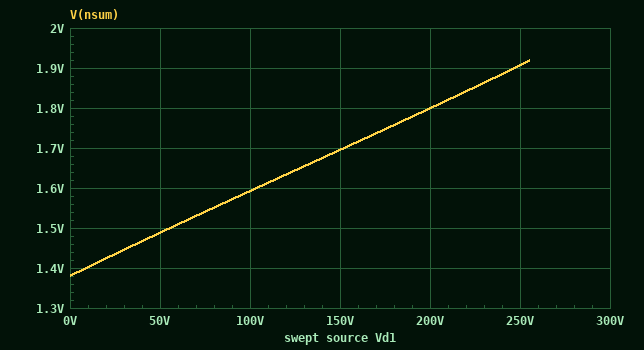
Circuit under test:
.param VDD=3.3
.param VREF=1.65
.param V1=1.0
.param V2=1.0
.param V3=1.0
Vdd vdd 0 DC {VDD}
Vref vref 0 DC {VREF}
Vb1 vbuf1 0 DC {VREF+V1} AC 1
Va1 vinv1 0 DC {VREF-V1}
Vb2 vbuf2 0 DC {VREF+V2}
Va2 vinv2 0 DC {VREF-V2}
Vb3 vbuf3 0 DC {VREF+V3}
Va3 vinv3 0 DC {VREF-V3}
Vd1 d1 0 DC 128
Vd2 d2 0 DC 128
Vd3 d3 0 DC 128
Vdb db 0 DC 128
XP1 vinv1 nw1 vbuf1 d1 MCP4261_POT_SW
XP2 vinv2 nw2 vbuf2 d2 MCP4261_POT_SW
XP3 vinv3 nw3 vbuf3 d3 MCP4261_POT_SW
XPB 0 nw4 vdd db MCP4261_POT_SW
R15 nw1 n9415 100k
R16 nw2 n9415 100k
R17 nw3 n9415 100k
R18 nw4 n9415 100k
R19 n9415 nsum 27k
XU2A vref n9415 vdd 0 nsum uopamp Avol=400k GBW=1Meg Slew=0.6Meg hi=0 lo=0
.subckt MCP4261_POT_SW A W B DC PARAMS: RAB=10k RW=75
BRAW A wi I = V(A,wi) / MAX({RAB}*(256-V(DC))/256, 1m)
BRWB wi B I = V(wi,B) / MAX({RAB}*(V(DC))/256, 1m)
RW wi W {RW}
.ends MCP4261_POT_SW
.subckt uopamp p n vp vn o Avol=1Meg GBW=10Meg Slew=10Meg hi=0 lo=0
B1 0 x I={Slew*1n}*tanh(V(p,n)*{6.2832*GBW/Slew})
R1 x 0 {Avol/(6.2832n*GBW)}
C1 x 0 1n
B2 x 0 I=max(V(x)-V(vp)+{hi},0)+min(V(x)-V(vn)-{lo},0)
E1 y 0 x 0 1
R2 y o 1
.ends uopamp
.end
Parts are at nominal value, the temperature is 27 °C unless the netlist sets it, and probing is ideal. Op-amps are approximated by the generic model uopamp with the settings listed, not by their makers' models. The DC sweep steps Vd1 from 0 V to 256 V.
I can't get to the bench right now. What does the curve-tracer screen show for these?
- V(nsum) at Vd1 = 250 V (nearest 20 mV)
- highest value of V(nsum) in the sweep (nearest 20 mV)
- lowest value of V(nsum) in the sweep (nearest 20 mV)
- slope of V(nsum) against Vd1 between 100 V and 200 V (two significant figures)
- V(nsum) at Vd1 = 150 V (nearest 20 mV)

1.90 V
1.92 V
1.38 V
0.0021 V/V
1.70 V
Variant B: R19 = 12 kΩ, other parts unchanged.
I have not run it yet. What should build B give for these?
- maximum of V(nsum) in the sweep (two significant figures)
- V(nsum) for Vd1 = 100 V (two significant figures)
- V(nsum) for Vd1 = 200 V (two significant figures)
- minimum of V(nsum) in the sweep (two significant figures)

1.8 V
1.6 V
1.7 V
1.5 V
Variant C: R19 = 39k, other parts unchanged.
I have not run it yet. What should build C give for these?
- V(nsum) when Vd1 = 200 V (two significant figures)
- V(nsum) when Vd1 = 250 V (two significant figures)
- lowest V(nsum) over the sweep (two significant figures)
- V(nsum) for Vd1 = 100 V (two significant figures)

1.9 V
2.0 V
1.3 V
1.6 V
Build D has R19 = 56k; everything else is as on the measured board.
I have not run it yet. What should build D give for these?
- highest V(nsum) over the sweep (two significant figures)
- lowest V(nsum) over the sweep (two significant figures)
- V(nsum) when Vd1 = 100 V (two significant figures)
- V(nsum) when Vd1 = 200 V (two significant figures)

2.2 V
1.1 V
1.5 V
2.0 V
